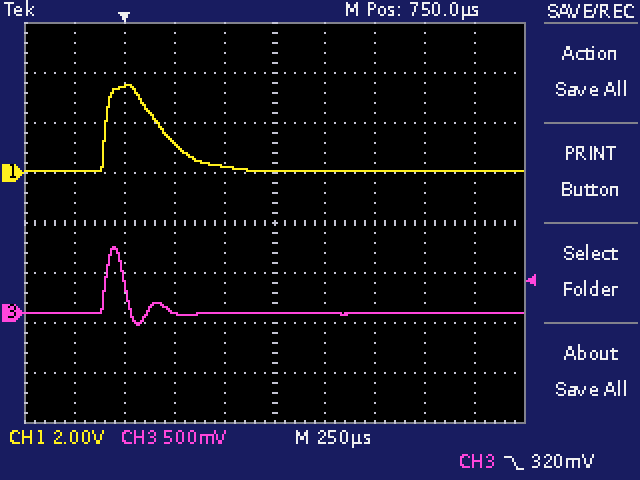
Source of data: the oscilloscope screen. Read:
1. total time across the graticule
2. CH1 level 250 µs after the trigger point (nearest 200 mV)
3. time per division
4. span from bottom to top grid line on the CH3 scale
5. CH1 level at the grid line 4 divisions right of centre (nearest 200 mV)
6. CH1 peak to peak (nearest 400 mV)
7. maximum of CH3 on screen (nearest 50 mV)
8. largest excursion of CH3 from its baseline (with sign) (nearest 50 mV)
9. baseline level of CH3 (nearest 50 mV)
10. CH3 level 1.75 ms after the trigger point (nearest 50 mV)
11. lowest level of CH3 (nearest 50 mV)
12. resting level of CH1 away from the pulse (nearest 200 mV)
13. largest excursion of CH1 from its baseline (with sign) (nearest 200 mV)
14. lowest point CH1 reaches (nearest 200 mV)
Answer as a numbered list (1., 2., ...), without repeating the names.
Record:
1. 2.5 ms
2. 1.2 V
3. 250 µs
4. 4 V
5. 0.0 V
6. 3.6 V
7. 650 mV
8. +650 mV
9. 0 mV
10. 0 mV
11. -100 mV
12. 0.0 V
13. +3.4 V
14. 0.0 V
